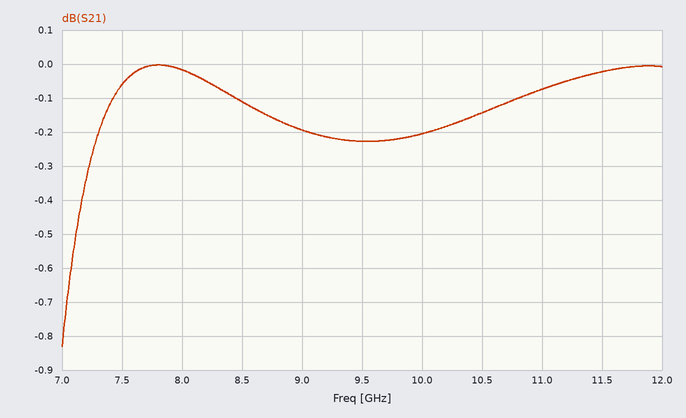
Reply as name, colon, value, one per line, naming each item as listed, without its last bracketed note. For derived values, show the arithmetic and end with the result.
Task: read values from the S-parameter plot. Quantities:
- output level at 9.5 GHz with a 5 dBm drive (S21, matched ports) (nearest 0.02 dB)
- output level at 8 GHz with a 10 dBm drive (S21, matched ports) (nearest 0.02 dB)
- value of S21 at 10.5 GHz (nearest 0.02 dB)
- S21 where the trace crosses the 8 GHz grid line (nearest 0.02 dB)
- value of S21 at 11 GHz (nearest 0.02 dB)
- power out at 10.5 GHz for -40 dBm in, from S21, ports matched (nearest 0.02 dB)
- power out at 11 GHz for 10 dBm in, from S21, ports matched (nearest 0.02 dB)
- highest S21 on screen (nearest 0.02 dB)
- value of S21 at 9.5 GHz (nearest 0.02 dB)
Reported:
output level at 9.5 GHz with a 5 dBm drive (S21, matched ports): 5 dBm + (-0.22 dB) = 4.78 dBm
output level at 8 GHz with a 10 dBm drive (S21, matched ports): 10 dBm + (-0.02 dB) = 9.98 dBm
value of S21 at 10.5 GHz: -0.14 dB
S21 where the trace crosses the 8 GHz grid line: -0.02 dB
value of S21 at 11 GHz: -0.08 dB
power out at 10.5 GHz for -40 dBm in, from S21, ports matched: -40 dBm + (-0.14 dB) = -40.14 dBm
power out at 11 GHz for 10 dBm in, from S21, ports matched: 10 dBm + (-0.08 dB) = 9.92 dBm
highest S21 on screen: 0.00 dB
value of S21 at 9.5 GHz: -0.22 dB
